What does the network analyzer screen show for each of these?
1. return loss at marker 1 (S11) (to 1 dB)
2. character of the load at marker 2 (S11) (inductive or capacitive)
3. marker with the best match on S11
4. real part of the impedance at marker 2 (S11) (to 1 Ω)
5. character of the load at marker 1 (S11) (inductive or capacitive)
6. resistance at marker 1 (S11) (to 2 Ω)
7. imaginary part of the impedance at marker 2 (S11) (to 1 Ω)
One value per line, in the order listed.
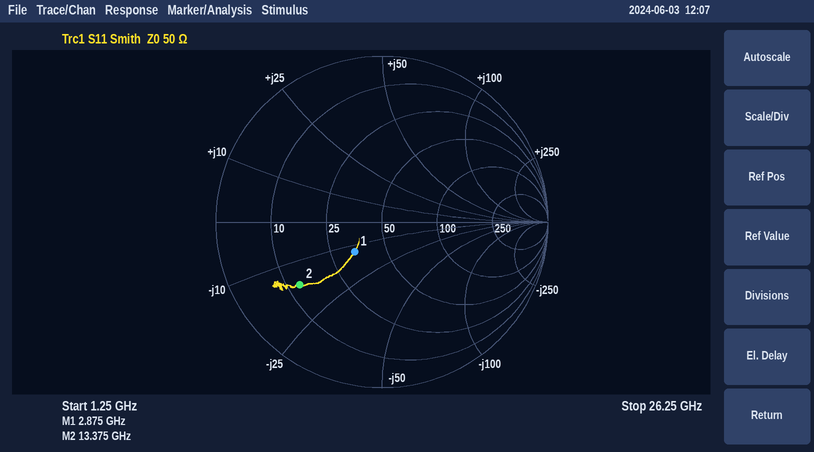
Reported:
12 dB
capacitive
marker 1
13 Ω
capacitive
34 Ω
-16 Ω
